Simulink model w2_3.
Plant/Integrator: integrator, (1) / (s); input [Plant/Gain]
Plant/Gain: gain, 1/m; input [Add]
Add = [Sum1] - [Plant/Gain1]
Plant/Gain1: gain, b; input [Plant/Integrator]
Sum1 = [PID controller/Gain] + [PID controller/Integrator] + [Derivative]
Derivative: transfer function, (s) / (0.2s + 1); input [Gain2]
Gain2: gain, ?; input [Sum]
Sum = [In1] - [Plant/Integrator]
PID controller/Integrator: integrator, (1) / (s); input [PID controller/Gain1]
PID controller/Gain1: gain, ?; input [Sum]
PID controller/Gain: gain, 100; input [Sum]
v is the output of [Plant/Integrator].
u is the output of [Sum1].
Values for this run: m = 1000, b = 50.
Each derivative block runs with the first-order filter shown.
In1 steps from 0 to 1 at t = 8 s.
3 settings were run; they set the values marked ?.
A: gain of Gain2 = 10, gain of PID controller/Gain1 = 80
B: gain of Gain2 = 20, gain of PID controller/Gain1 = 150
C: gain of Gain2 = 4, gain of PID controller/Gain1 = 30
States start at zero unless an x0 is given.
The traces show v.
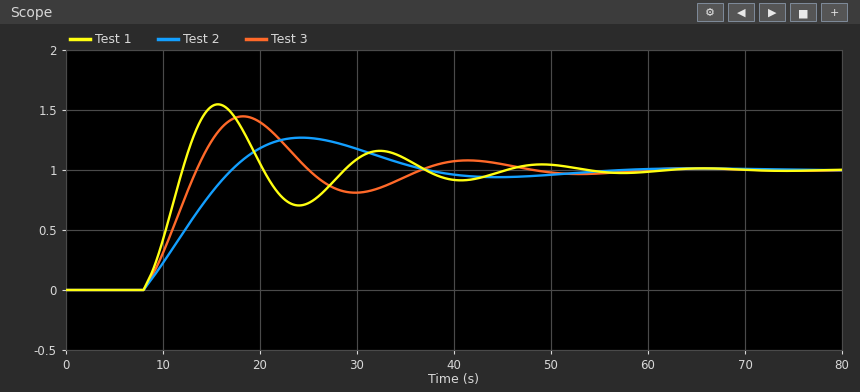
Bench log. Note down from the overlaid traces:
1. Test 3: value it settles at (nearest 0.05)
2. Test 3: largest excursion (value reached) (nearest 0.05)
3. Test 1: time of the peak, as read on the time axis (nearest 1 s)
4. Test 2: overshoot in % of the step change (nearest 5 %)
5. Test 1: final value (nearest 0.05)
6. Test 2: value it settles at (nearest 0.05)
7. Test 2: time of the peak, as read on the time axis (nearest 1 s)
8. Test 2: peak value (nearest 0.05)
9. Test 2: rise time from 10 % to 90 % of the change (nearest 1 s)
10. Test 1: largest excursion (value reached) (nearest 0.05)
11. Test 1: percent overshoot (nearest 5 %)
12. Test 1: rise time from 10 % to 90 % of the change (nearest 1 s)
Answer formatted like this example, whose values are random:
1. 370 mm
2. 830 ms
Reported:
1. 1.00
2. 1.45
3. 16 s
4. 25 %
5. 1.00
6. 1.00
7. 24 s
8. 1.25
9. 7 s
10. 1.55
11. 55 %
12. 3 s
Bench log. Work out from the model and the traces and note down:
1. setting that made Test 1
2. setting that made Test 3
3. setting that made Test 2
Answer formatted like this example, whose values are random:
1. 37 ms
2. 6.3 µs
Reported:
1. B
2. A
3. C
